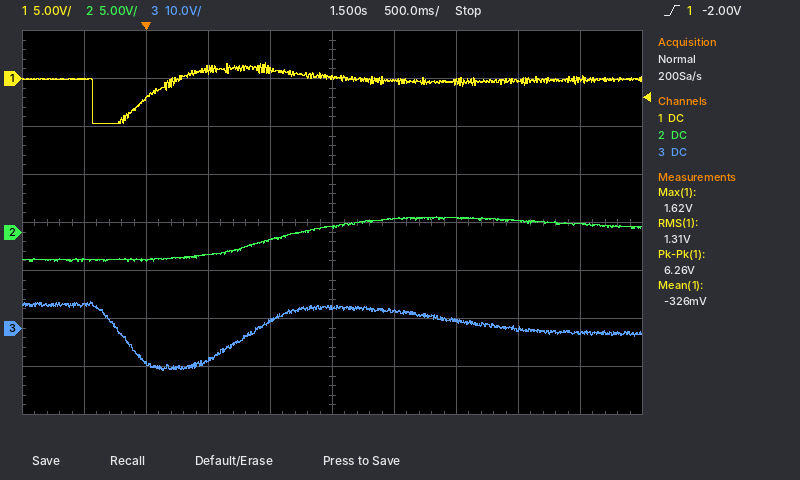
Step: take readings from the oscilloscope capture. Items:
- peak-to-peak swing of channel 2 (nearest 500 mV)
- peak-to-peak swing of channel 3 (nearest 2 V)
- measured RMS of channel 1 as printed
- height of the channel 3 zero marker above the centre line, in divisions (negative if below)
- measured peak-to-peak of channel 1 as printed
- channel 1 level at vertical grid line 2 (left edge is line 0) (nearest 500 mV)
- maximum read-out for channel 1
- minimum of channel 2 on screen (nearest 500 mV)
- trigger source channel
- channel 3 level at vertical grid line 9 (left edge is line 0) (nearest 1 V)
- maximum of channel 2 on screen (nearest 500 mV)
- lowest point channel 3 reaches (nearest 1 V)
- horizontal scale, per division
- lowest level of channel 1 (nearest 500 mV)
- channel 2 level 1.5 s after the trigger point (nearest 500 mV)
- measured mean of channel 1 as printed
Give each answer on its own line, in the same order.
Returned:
4.5 V
14 V
1.31 V
-2.2 div
6.26 V
-2.0 V
1.62 V
-3.0 V
channel 1
-1 V
1.5 V
-9 V
500 ms
-4.5 V
500 mV
-326 mV
